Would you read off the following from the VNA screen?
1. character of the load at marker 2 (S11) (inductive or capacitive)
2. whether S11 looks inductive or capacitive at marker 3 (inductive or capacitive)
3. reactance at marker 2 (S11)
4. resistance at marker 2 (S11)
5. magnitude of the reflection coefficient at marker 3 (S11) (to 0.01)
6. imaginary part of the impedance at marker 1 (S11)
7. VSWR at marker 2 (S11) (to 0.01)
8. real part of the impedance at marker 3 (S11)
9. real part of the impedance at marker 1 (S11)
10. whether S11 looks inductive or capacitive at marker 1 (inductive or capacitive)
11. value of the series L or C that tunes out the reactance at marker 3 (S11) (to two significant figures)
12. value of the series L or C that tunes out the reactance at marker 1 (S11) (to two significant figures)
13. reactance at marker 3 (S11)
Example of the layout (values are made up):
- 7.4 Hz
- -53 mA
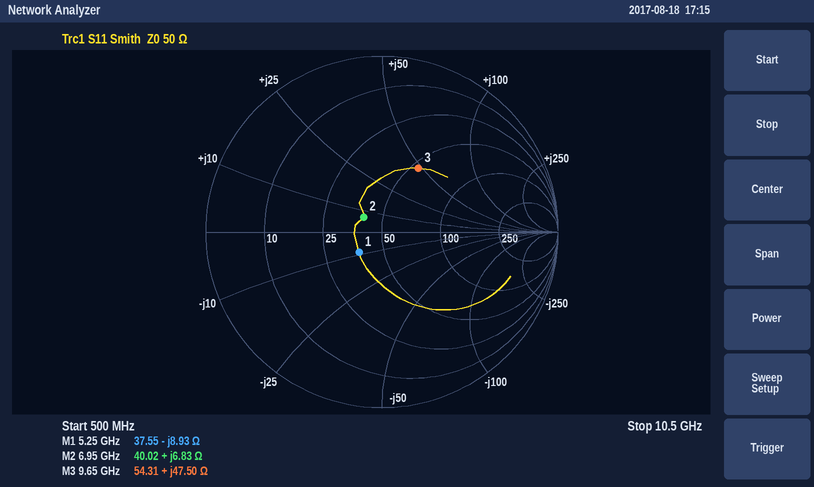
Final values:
- inductive
- inductive
- +6.83 Ω
- 40.02 Ω
- 0.42
- -8.93 Ω
- 1.31
- 54.31 Ω
- 37.55 Ω
- capacitive
- 350 fF
- 270 pH
- +47.50 Ω
